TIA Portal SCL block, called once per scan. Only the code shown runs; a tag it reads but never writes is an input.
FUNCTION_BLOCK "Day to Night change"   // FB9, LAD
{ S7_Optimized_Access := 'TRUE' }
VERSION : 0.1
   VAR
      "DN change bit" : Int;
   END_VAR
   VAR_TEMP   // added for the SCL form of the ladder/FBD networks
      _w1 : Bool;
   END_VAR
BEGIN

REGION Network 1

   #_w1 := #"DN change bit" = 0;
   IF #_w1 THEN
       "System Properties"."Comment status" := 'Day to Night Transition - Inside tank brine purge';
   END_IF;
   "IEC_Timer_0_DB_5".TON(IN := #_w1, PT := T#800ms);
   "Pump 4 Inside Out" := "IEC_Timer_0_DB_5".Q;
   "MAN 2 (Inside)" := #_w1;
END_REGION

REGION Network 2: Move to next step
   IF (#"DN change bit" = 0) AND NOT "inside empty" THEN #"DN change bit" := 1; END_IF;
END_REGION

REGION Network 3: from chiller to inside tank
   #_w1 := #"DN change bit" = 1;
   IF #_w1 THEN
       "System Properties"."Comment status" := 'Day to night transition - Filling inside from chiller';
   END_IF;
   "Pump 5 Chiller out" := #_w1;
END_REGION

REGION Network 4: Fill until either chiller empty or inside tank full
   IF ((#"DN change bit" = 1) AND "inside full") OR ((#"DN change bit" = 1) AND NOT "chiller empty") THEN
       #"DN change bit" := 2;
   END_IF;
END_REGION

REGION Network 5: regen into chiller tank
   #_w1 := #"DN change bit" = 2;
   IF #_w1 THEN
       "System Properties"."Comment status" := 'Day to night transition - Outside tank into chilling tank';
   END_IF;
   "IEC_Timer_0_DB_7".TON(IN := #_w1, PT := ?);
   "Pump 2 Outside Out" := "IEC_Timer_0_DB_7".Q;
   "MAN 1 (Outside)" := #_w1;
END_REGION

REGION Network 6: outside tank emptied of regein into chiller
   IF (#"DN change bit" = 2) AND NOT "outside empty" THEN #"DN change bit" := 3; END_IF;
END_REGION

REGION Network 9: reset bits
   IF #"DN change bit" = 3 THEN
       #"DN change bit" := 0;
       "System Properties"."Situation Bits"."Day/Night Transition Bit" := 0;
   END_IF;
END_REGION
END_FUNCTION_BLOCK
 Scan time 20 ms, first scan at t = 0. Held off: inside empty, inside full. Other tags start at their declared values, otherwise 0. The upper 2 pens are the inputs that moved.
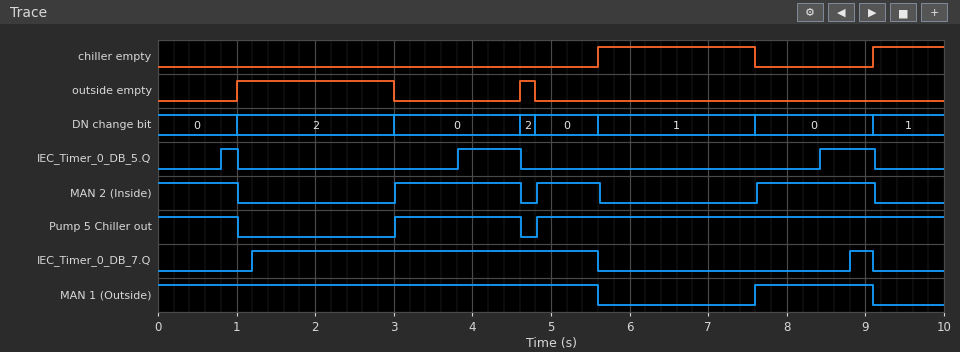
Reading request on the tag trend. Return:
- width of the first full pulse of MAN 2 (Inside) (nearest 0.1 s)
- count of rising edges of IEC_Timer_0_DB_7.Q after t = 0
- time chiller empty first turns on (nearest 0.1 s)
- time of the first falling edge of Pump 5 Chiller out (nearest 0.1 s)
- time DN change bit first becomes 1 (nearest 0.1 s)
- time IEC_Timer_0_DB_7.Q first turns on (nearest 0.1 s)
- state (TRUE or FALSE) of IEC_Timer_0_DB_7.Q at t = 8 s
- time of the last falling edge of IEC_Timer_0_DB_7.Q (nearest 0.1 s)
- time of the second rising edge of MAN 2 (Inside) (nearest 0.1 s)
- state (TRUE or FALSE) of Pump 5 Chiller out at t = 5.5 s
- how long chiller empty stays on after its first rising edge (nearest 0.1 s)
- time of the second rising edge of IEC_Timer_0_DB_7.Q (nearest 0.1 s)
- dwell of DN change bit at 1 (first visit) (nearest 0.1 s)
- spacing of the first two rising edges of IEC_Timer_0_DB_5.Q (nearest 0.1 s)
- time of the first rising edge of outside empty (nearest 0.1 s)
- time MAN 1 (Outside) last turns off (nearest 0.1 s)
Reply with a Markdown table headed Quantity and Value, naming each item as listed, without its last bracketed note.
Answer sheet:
| Quantity | Value |
|---|---|
| width of the first full pulse of MAN 2 (Inside) | 1.6 s |
| count of rising edges of IEC_Timer_0_DB_7.Q after t = 0 | 2 |
| time chiller empty first turns on | 5.6 s |
| time of the first falling edge of Pump 5 Chiller out | 1.0 s |
| time DN change bit first becomes 1 | 5.6 s |
| time IEC_Timer_0_DB_7.Q first turns on | 1.2 s |
| state (TRUE or FALSE) of IEC_Timer_0_DB_7.Q at t = 8 s | FALSE |
| time of the last falling edge of IEC_Timer_0_DB_7.Q | 9.1 s |
| time of the second rising edge of MAN 2 (Inside) | 4.8 s |
| state (TRUE or FALSE) of Pump 5 Chiller out at t = 5.5 s | TRUE |
| how long chiller empty stays on after its first rising edge | 2.0 s |
| time of the second rising edge of IEC_Timer_0_DB_7.Q | 8.8 s |
| dwell of DN change bit at 1 (first visit) | 2.0 s |
| spacing of the first two rising edges of IEC_Timer_0_DB_5.Q | 3.0 s |
| time of the first rising edge of outside empty | 1.0 s |
| time MAN 1 (Outside) last turns off | 9.1 s |
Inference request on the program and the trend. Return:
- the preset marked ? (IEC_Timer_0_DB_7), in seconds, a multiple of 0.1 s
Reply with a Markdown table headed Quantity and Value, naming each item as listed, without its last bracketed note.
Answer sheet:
| Quantity | Value |
|---|---|
| the preset marked ? (IEC_Timer_0_DB_7), in seconds, a multiple of 0.1 s | 1.2 s |
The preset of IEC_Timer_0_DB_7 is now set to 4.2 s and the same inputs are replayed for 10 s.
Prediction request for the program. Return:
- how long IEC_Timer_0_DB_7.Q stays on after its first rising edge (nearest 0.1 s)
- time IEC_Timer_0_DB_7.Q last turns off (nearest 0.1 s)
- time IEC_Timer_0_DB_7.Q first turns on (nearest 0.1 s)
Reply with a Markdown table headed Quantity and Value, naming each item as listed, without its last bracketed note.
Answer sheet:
| Quantity | Value |
|---|---|
| how long IEC_Timer_0_DB_7.Q stays on after its first rising edge | 1.4 s |
| time IEC_Timer_0_DB_7.Q last turns off | 5.6 s |
| time IEC_Timer_0_DB_7.Q first turns on | 4.2 s |
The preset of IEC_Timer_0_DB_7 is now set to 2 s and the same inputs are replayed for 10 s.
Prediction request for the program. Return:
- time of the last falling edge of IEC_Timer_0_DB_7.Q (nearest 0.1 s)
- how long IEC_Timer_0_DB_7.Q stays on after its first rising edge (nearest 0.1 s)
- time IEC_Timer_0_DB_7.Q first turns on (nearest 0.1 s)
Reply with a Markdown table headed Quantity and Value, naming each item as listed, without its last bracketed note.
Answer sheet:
| Quantity | Value |
|---|---|
| time of the last falling edge of IEC_Timer_0_DB_7.Q | 5.6 s |
| how long IEC_Timer_0_DB_7.Q stays on after its first rising edge | 3.6 s |
| time IEC_Timer_0_DB_7.Q first turns on | 2.0 s |
